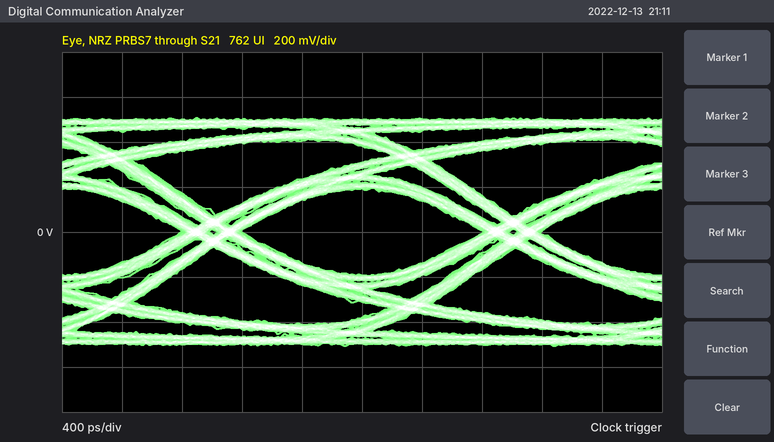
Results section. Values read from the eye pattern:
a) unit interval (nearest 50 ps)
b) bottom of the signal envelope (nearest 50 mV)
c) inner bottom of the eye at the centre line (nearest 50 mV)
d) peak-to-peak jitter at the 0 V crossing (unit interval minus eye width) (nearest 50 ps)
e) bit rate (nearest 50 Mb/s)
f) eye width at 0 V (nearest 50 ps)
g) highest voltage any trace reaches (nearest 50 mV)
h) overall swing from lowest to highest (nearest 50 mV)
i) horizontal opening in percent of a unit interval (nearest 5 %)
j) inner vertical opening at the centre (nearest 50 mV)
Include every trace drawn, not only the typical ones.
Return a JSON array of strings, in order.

["2.00 ns", "-500 mV", "-200 mV", "400 ps", "500 Mb/s", "1.60 ns", "500 mV", "1.00 V", "80 %", "400 mV"]
